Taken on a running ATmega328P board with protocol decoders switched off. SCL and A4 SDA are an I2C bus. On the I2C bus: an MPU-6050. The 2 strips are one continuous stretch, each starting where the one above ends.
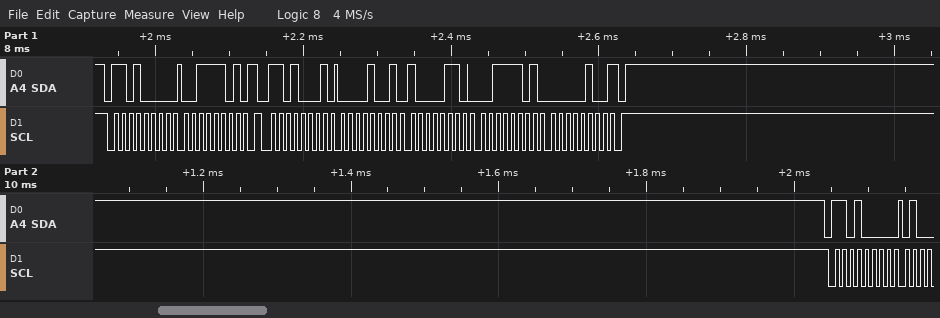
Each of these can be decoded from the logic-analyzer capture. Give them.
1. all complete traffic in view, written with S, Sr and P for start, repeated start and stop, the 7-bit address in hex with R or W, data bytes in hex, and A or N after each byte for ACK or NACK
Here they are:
S 68W A 3D A Sr 68R A 09 A 86 A 3D A 04 N P S 68W A
